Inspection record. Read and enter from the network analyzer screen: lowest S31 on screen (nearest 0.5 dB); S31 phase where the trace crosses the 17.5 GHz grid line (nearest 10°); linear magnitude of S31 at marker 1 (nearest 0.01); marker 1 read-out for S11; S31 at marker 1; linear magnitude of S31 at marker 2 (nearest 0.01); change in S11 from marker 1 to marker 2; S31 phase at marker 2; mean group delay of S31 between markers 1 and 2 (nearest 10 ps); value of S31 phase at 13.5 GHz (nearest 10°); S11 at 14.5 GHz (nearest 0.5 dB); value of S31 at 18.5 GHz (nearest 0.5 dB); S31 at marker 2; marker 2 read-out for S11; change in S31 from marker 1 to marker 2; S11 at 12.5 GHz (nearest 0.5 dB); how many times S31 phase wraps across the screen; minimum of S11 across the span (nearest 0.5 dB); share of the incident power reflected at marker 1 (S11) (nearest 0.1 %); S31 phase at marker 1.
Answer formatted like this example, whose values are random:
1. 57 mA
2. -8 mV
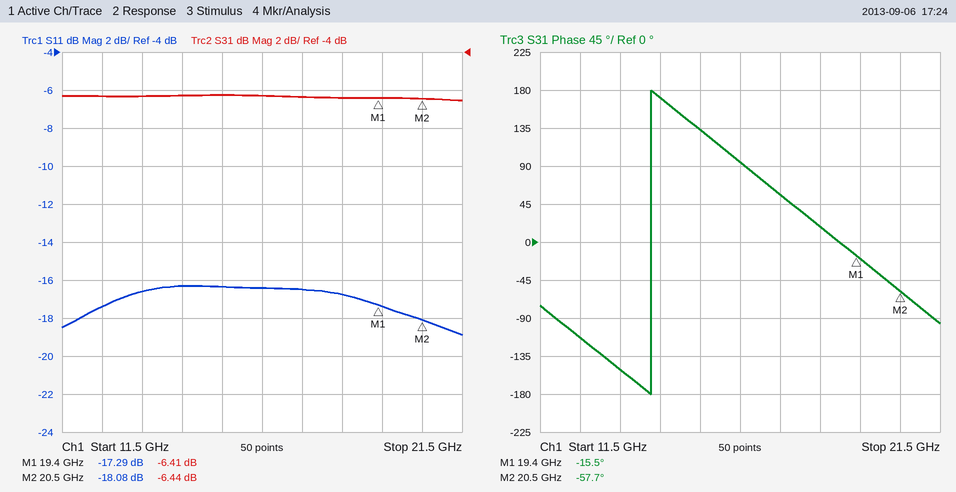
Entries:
1. -6.5 dB
2. 60°
3. 0.48
4. -17.29 dB
5. -6.41 dB
6. 0.48
7. -0.79 dB
8. -57.7°
9. 110 ps
10. -150°
11. -16.5 dB
12. -6.5 dB
13. -6.44 dB
14. -18.08 dB
15. -0.03 dB
16. -17.5 dB
17. 1
18. -19.0 dB
19. 1.9 %
20. -15.5°
